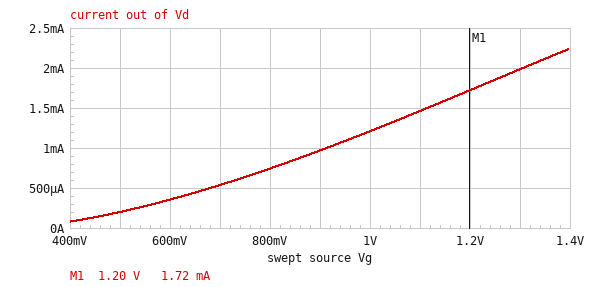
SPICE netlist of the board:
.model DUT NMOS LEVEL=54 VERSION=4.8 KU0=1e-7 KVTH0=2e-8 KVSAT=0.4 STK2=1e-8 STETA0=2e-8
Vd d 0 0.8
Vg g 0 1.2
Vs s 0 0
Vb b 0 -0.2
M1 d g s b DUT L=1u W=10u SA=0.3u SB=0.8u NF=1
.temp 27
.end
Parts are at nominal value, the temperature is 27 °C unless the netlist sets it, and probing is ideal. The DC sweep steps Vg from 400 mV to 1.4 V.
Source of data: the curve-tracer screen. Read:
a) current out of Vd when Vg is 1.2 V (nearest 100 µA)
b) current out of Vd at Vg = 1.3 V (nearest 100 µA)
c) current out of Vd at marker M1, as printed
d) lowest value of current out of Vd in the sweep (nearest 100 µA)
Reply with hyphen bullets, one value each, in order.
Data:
- 1.7 mA
- 2.0 mA
- 1.72 mA
- 100 µA
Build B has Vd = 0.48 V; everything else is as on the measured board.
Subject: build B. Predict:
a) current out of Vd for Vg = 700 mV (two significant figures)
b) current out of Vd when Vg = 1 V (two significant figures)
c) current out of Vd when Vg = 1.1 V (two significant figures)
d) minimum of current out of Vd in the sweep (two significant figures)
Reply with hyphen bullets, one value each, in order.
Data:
- 510 µA
- 1.1 mA
- 1.3 mA
- 77 µA
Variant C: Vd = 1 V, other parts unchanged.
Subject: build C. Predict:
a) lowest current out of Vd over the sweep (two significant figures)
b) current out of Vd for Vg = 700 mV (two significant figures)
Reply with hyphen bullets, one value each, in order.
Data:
- 83 µA
- 550 µA
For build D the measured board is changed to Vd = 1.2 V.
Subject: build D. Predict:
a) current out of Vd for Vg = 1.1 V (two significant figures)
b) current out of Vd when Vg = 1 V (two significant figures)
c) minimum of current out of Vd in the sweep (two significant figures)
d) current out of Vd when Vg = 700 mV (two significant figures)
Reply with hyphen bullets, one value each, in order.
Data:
- 1.5 mA
- 1.3 mA
- 85 µA
- 560 µA
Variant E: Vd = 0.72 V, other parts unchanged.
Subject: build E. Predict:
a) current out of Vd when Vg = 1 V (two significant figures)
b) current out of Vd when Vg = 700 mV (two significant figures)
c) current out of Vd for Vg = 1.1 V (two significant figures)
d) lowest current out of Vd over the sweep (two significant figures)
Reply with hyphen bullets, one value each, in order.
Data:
- 1.2 mA
- 530 µA
- 1.4 mA
- 80 µA
